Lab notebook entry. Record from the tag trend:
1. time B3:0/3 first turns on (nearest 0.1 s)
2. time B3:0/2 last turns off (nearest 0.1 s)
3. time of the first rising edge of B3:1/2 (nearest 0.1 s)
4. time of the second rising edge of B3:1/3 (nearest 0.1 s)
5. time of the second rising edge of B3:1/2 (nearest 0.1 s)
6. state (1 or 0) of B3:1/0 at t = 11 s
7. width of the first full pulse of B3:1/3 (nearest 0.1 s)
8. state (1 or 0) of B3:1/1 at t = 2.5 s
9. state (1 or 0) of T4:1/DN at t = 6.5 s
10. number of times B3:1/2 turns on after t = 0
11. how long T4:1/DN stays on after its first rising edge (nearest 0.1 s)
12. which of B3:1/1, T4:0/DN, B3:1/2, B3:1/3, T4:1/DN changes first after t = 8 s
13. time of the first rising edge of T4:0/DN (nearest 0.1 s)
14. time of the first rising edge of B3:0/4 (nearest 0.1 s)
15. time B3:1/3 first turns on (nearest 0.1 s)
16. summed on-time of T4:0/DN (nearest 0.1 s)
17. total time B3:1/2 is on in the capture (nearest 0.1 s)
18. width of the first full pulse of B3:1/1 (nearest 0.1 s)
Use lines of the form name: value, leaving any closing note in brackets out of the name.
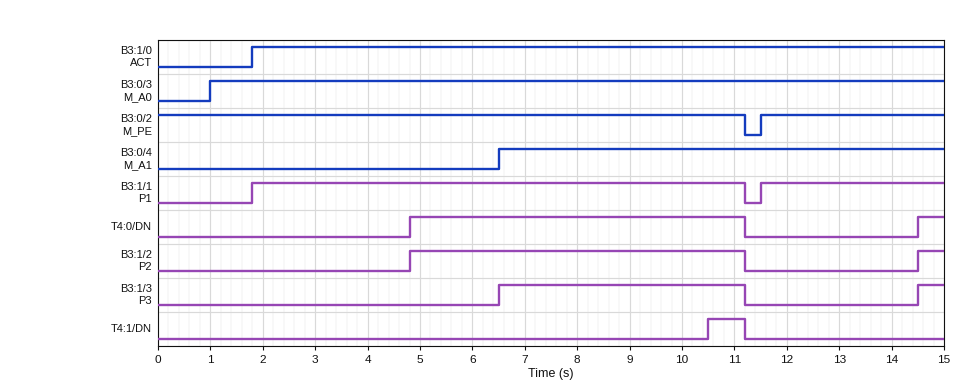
time B3:0/3 first turns on: 1.0 s
time B3:0/2 last turns off: 11.2 s
time of the first rising edge of B3:1/2: 4.8 s
time of the second rising edge of B3:1/3: 14.5 s
time of the second rising edge of B3:1/2: 14.5 s
state (1 or 0) of B3:1/0 at t = 11 s: 1
width of the first full pulse of B3:1/3: 4.7 s
state (1 or 0) of B3:1/1 at t = 2.5 s: 1
state (1 or 0) of T4:1/DN at t = 6.5 s: 0
number of times B3:1/2 turns on after t = 0: 2
how long T4:1/DN stays on after its first rising edge: 0.7 s
which of B3:1/1, T4:0/DN, B3:1/2, B3:1/3, T4:1/DN changes first after t = 8 s: T4:1/DN
time of the first rising edge of T4:0/DN: 4.8 s
time of the first rising edge of B3:0/4: 6.5 s
time B3:1/3 first turns on: 6.5 s
summed on-time of T4:0/DN: 6.9 s
total time B3:1/2 is on in the capture: 6.9 s
width of the first full pulse of B3:1/1: 9.4 s
